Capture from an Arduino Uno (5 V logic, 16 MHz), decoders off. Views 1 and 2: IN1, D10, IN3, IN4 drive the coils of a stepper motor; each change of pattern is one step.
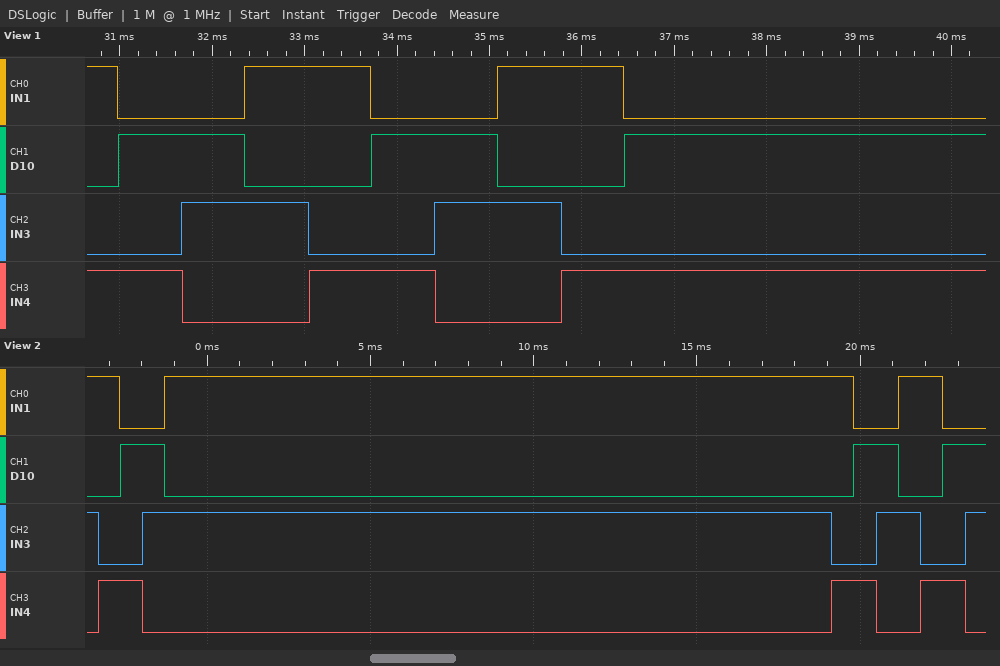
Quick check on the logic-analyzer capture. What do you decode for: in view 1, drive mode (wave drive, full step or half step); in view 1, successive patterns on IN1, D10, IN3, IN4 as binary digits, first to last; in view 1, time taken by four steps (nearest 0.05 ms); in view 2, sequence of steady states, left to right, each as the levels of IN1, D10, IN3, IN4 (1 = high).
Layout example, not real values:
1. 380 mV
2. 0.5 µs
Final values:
1. full step
2. 1001 0101 0110 1010 1001 0101 0110 1010 1001 0101
3. 2.75 ms
4. 1010 1001 0101 0110 1010 1001 0101 0110 1010 1001 0101 0110
